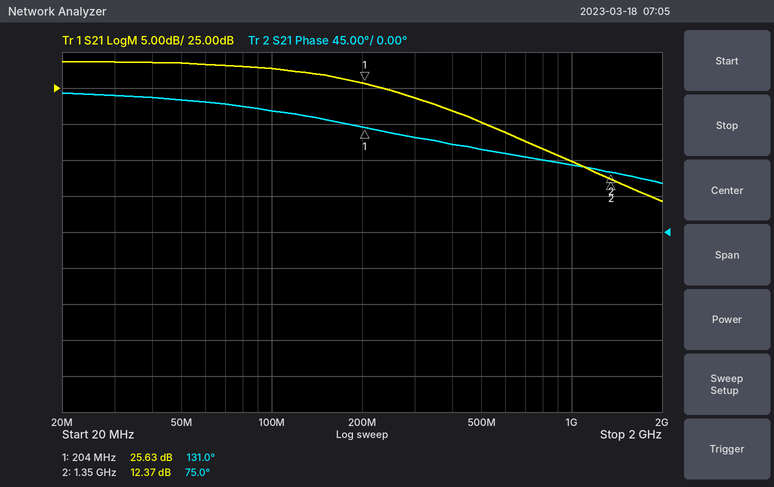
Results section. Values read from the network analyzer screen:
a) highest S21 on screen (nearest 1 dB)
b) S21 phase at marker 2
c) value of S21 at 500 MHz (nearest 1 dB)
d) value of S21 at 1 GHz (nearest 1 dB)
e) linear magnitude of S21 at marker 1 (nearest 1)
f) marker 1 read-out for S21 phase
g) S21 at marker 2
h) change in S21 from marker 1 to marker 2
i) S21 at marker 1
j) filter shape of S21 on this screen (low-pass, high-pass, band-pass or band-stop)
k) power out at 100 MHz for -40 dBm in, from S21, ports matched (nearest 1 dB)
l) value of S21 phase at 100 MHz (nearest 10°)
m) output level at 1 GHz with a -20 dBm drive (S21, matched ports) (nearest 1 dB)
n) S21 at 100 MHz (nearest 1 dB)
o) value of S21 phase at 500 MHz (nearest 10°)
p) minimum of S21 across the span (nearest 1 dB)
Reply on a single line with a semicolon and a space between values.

29 dB; 75.0°; 20 dB; 15 dB; 19; 131.0°; 12.37 dB; -13.26 dB; 25.63 dB; low-pass; -12 dBm; 150°; -5 dBm; 28 dB; 100°; 9 dB
